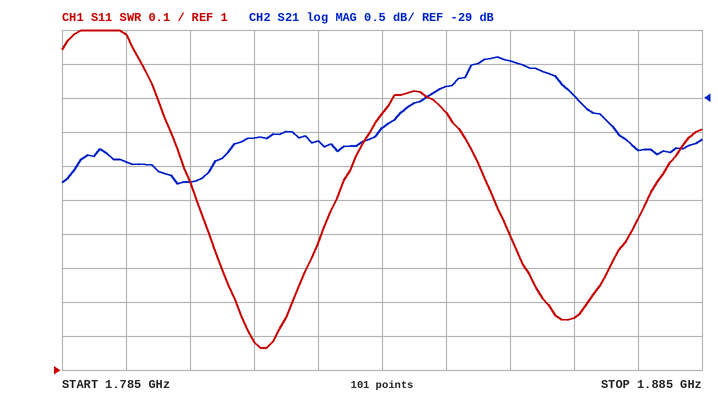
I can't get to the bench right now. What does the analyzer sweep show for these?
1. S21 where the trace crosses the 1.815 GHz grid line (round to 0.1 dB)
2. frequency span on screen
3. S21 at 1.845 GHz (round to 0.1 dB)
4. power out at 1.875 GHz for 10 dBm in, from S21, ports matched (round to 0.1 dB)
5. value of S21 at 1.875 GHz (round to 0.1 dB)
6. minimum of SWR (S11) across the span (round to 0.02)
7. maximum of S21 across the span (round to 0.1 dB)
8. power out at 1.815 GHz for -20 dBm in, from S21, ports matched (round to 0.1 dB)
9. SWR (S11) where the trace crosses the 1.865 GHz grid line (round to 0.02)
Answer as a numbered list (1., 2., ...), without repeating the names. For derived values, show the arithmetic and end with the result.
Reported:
1. -29.6 dB
2. 100 MHz
3. -28.8 dB
4. 10 dBm + (-29.8 dB) = -19.8 dBm
5. -29.8 dB
6. 1.06
7. -28.4 dB
8. -20 dBm + (-29.6 dB) = -49.6 dBm
9. 1.16
